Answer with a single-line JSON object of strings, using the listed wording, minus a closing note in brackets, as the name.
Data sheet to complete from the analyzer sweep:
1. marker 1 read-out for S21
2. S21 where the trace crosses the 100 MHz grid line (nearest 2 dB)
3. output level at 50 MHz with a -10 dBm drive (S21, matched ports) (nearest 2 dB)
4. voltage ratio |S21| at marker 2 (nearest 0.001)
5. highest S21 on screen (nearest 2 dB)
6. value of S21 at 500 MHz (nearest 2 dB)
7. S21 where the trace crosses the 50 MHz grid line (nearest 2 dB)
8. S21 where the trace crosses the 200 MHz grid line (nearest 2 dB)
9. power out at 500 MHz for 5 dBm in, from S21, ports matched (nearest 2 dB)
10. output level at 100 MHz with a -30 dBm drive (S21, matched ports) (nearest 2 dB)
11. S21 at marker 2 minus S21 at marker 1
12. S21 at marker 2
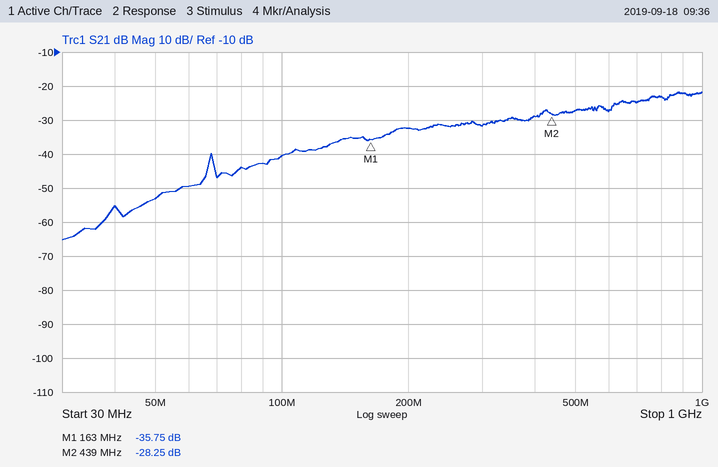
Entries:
{"marker 1 read-out for S21": "-35.75 dB", "S21 where the trace crosses the 100 MHz grid line": "-40 dB", "output level at 50 MHz with a -10 dBm drive (S21, matched ports)": "-64 dBm", "voltage ratio |S21| at marker 2": "0.039", "highest S21 on screen": "-22 dB", "value of S21 at 500 MHz": "-28 dB", "S21 where the trace crosses the 50 MHz grid line": "-54 dB", "S21 where the trace crosses the 200 MHz grid line": "-32 dB", "power out at 500 MHz for 5 dBm in, from S21, ports matched": "-22 dBm", "output level at 100 MHz with a -30 dBm drive (S21, matched ports)": "-70 dBm", "S21 at marker 2 minus S21 at marker 1": "7.50 dB", "S21 at marker 2": "-28.25 dB"}
